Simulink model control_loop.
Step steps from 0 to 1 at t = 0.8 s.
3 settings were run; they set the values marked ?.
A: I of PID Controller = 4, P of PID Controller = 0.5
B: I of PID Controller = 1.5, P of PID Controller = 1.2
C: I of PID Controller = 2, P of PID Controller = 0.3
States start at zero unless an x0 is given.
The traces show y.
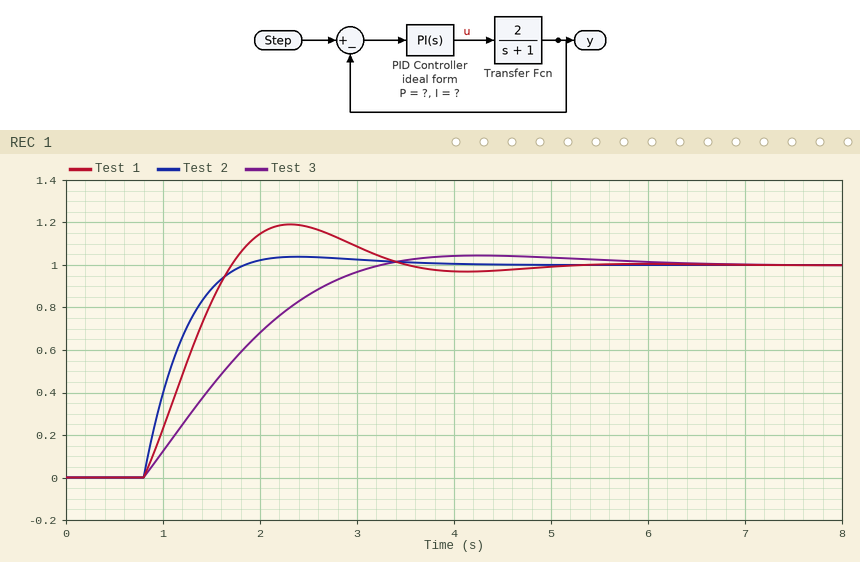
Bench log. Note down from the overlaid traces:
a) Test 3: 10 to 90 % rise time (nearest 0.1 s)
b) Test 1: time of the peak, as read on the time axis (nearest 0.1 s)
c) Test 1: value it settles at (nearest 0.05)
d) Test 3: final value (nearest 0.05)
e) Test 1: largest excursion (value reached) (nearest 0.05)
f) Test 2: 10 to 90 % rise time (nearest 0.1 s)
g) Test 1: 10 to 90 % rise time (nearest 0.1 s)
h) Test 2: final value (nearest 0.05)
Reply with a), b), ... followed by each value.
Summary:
a) 1.7 s
b) 2.3 s
c) 1.00
d) 1.00
e) 1.20
f) 0.7 s
g) 0.7 s
h) 1.00
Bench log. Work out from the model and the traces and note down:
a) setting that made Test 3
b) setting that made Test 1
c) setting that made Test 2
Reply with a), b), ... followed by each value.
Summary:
a) C
b) A
c) B
